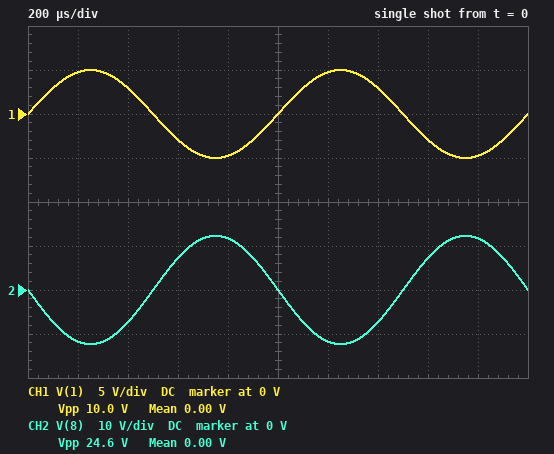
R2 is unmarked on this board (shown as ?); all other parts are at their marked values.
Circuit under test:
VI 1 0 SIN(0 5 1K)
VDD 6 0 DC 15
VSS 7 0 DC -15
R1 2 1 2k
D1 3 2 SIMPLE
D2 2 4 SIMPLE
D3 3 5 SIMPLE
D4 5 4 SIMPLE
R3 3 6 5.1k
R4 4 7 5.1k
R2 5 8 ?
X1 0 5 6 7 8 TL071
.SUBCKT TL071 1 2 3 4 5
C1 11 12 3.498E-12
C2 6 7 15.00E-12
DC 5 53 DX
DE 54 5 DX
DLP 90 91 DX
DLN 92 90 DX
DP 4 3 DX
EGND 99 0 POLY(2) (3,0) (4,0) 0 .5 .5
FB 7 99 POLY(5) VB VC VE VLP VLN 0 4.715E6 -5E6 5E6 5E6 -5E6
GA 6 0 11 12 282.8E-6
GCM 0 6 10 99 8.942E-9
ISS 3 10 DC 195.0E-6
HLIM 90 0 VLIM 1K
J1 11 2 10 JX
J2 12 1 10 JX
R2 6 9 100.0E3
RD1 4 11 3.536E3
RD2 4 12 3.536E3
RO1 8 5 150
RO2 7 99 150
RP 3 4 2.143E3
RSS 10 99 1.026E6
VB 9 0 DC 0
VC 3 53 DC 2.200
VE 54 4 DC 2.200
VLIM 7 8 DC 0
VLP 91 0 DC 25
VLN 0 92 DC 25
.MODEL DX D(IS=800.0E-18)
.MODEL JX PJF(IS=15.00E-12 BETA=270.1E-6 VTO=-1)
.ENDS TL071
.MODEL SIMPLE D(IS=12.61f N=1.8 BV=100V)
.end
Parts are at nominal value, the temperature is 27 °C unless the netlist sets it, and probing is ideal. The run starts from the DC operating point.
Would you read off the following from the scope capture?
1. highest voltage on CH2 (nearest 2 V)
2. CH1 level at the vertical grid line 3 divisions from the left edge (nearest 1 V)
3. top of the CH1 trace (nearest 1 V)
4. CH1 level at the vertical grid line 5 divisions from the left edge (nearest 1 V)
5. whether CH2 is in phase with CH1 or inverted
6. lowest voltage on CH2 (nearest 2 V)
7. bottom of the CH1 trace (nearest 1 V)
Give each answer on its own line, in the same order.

12 V
-3 V
5 V
0 V
inverted
-12 V
-5 V
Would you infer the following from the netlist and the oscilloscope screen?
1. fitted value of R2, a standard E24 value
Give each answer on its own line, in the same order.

5.1 kΩ
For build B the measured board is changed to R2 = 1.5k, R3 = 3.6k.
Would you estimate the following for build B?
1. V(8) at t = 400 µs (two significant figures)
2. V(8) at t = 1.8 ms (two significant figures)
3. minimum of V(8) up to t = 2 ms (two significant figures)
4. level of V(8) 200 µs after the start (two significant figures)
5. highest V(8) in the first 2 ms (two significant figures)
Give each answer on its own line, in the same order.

-3.8 V
1.8 V
-5.3 V
-5.1 V
2.0 V
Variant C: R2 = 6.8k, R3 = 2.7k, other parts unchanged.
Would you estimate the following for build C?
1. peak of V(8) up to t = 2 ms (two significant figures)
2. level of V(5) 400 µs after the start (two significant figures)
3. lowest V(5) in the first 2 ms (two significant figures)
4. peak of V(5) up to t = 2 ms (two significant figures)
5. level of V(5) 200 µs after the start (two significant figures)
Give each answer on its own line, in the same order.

530 mV
1.5 V
-13 mV
2.4 V
2.3 V
